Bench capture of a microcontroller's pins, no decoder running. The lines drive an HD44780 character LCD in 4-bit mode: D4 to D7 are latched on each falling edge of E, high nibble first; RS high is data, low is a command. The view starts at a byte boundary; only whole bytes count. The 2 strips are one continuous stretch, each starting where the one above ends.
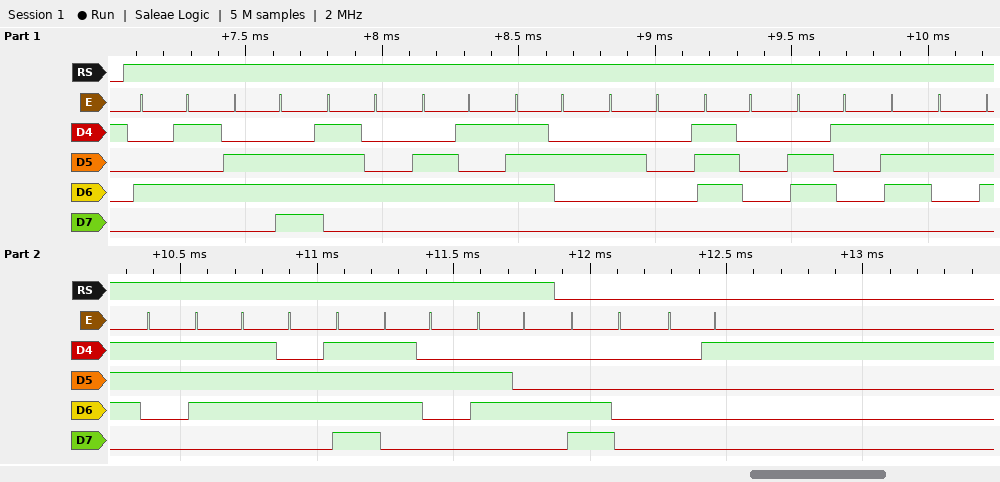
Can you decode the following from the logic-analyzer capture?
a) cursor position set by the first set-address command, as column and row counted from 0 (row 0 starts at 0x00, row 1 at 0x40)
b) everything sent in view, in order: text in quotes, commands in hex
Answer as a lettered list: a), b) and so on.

a) column 0, row 1
b) "Enter password" 0xC0 0x01
